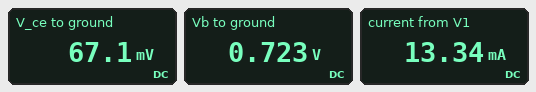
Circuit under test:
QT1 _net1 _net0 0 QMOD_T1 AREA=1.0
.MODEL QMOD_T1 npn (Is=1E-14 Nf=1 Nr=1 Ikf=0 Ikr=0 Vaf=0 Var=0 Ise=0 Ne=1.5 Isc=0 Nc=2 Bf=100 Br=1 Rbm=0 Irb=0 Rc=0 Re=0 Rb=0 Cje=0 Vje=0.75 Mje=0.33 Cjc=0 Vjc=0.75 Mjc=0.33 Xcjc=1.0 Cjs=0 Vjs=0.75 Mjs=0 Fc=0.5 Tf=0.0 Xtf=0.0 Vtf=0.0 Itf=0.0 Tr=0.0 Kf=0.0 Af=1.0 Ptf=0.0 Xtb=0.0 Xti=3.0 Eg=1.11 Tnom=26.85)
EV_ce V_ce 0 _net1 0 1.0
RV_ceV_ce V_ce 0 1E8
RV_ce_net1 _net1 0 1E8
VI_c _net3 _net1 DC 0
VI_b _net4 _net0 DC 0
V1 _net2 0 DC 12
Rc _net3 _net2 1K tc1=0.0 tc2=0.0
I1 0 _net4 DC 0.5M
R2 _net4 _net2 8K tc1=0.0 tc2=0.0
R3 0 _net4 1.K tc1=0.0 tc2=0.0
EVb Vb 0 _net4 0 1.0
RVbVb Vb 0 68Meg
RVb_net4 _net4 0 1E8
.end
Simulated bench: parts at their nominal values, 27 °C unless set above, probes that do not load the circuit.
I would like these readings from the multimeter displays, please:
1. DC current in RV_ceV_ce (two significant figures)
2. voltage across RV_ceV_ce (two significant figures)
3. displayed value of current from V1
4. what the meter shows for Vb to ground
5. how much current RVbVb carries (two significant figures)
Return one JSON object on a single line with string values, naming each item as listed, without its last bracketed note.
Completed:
{"DC current in RV_ceV_ce": "670 pA", "voltage across RV_ceV_ce": "67 mV", "displayed value of current from V1": "13.34 mA", "what the meter shows for Vb to ground": "0.723 V", "how much current RVbVb carries": "11 nA"}
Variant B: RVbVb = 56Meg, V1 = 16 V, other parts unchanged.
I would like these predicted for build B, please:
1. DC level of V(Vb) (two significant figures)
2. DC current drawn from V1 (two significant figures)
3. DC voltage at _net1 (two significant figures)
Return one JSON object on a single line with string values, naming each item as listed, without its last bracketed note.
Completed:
{"DC level of V(Vb)": "730 mV", "DC current drawn from V1": "18 mA", "DC voltage at _net1": "66 mV"}
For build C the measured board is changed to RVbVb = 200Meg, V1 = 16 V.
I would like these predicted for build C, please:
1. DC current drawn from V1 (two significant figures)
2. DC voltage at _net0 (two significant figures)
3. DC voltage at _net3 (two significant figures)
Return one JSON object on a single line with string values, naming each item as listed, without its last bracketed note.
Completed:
{"DC current drawn from V1": "18 mA", "DC voltage at _net0": "730 mV", "DC voltage at _net3": "66 mV"}
